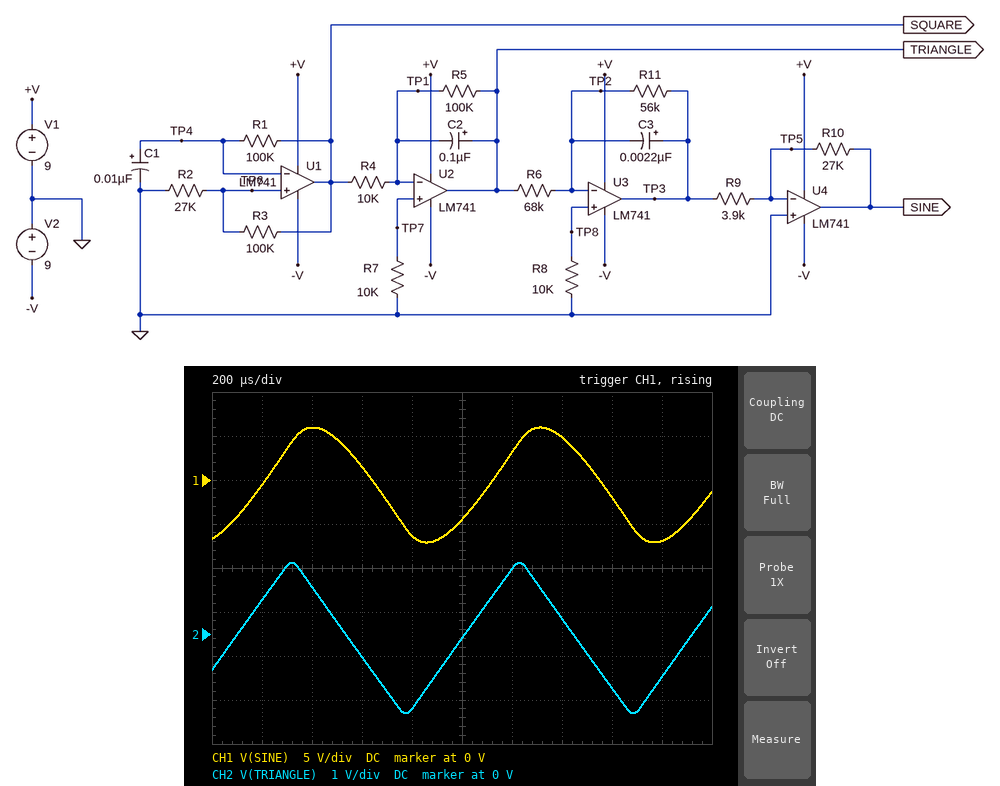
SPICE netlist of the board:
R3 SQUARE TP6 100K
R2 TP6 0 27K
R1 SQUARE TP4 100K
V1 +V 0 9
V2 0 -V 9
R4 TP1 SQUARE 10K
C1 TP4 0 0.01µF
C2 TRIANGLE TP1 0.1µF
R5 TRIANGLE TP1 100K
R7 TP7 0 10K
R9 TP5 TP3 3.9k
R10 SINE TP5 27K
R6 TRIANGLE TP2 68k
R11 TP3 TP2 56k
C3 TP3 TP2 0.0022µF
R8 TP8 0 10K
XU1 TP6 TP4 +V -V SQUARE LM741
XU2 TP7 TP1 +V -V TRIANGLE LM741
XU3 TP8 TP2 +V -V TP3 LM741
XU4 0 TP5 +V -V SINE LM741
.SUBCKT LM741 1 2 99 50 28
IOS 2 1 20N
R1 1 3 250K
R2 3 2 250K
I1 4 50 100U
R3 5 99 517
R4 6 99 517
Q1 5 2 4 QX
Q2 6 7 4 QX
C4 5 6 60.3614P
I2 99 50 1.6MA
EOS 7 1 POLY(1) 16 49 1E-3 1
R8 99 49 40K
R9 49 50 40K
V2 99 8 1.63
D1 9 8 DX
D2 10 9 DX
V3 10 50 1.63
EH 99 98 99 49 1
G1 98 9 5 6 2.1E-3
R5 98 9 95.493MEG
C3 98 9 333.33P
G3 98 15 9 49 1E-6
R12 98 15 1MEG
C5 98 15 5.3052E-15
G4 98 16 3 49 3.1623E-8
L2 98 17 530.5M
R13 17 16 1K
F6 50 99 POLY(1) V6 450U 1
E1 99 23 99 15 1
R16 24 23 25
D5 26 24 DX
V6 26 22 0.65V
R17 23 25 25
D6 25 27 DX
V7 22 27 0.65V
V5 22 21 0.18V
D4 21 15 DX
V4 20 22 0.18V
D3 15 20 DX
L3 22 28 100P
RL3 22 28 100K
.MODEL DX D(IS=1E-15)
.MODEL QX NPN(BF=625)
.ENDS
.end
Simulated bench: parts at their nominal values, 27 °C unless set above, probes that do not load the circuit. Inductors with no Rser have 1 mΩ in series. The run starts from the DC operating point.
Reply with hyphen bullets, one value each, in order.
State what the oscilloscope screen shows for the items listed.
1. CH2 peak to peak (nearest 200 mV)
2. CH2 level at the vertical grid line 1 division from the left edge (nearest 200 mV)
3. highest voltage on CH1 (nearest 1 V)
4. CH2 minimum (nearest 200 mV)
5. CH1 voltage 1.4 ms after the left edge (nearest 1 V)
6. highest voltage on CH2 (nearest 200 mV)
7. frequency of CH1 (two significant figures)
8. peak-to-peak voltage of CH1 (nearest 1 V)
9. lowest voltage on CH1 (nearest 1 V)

- 3.4 V
- 800 mV
- 6 V
- -1.8 V
- 5 V
- 1.6 V
- 1.1 kHz
- 13 V
- -7 V
